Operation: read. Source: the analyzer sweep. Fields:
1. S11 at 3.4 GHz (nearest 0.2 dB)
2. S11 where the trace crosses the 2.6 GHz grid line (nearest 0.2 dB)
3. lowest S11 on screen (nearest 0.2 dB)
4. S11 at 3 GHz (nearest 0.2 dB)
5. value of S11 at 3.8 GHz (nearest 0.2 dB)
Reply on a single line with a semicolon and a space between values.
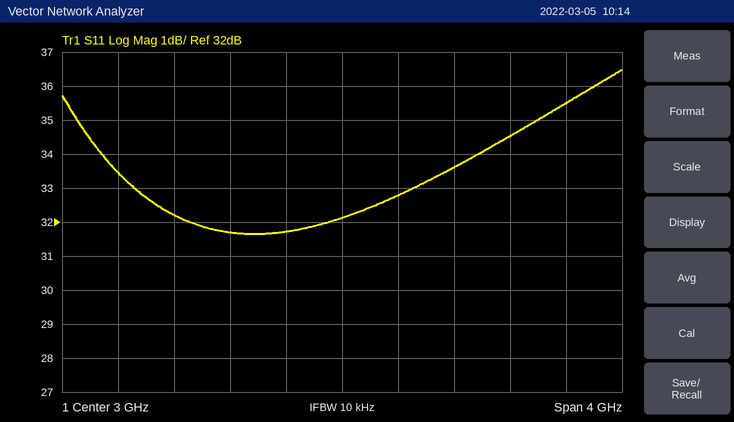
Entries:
32.8 dB; 31.8 dB; 31.6 dB; 32.2 dB; 33.6 dB
